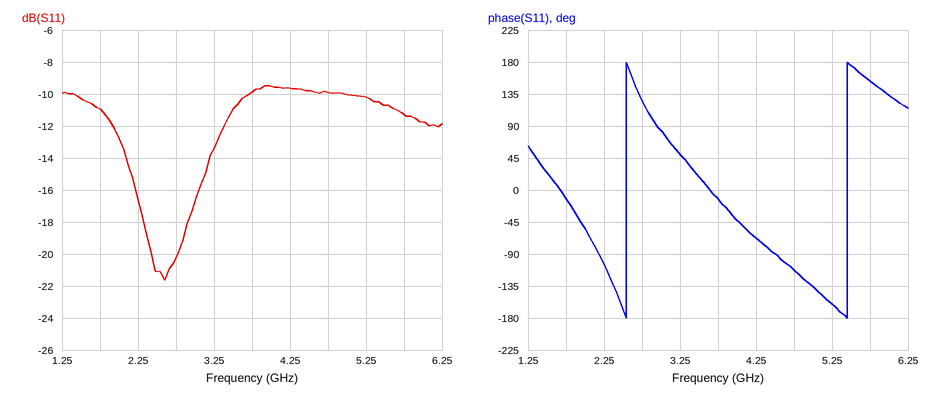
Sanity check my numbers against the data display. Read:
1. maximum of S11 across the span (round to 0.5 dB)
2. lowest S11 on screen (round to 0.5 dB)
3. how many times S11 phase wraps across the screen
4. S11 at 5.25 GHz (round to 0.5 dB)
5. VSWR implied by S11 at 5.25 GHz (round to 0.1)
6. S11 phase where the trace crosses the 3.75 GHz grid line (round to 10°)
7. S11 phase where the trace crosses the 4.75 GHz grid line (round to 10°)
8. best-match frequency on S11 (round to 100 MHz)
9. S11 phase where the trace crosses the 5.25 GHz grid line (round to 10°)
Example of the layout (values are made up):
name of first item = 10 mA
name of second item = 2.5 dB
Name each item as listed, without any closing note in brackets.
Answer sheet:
maximum of S11 across the span = -9.5 dB
lowest S11 on screen = -21.5 dB
how many times S11 phase wraps across the screen = 2
S11 at 5.25 GHz = -10.0 dB
VSWR implied by S11 at 5.25 GHz = 1.9
S11 phase where the trace crosses the 3.75 GHz grid line = -10°
S11 phase where the trace crosses the 4.75 GHz grid line = -110°
best-match frequency on S11 = 2.6 GHz
S11 phase where the trace crosses the 5.25 GHz grid line = -160°
